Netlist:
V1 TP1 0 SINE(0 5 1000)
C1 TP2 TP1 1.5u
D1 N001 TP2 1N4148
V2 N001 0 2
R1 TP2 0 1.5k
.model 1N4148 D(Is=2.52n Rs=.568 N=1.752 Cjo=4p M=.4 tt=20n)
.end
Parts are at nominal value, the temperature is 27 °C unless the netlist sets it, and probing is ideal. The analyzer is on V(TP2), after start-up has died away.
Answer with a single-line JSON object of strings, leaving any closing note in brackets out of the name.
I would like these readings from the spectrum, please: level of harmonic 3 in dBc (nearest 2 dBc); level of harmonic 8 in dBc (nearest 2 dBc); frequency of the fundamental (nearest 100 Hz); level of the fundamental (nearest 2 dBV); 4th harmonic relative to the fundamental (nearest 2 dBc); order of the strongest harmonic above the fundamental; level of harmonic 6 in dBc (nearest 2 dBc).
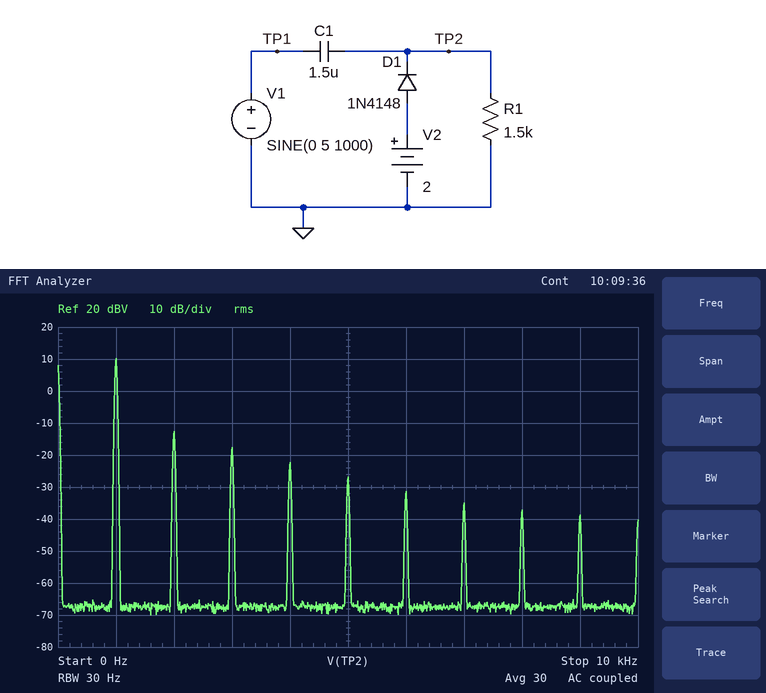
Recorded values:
{"level of harmonic 3 in dBc": "-28 dBc", "level of harmonic 8 in dBc": "-48 dBc", "frequency of the fundamental": "1.0 kHz", "level of the fundamental": "10 dBV", "4th harmonic relative to the fundamental": "-32 dBc", "order of the strongest harmonic above the fundamental": "2", "level of harmonic 6 in dBc": "-42 dBc"}
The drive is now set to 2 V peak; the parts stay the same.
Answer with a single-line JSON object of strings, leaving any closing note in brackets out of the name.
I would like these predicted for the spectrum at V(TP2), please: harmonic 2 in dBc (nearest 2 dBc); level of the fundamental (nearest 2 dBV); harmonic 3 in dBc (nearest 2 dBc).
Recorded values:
{"harmonic 2 in dBc": "-20 dBc", "level of the fundamental": "2 dBV", "harmonic 3 in dBc": "-26 dBc"}
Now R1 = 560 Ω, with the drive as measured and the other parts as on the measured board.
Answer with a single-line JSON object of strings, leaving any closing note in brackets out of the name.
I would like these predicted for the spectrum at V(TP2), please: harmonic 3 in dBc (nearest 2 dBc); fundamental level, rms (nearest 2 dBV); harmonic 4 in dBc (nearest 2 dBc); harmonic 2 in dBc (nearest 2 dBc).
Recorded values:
{"harmonic 3 in dBc": "-24 dBc", "fundamental level, rms": "8 dBV", "harmonic 4 in dBc": "-30 dBc", "harmonic 2 in dBc": "-16 dBc"}
